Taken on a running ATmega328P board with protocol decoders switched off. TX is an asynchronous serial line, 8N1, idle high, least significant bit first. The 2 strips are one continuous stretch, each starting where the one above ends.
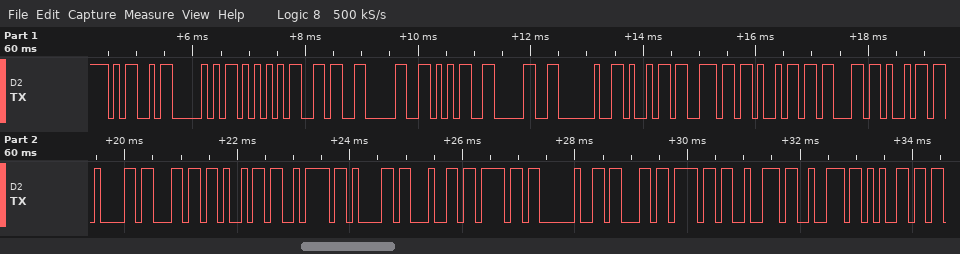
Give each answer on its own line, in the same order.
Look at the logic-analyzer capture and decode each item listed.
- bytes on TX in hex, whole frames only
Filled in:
4D 50 55 36 30 35 30 20 69 6E 69 63 69 61 6C 69 7A 61 64 6F 20 63 6F 72 72 65
